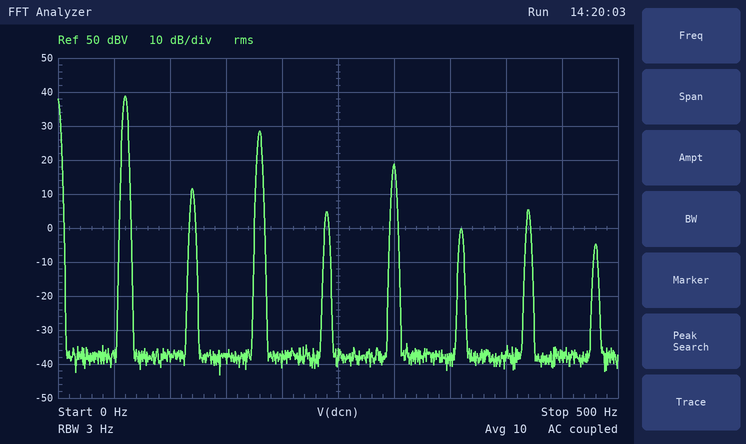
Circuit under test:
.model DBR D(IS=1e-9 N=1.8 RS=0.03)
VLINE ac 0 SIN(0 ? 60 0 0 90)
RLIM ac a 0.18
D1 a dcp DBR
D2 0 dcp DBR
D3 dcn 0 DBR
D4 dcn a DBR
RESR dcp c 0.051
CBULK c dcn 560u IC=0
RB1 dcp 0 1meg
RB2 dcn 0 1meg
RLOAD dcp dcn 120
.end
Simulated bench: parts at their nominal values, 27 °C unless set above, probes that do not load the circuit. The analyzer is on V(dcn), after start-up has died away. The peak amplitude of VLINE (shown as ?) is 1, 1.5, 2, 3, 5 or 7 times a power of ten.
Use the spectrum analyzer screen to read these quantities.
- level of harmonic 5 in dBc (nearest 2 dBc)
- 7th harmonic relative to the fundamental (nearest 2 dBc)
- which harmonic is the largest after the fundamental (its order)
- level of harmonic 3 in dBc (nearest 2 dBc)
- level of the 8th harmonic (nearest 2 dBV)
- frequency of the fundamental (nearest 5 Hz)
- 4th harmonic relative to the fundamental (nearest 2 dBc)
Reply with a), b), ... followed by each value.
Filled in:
a) -20 dBc
b) -34 dBc
c) 3
d) -10 dBc
e) -4 dBV
f) 60 Hz
g) -34 dBc
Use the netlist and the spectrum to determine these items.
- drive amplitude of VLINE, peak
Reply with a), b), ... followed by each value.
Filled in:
a) 300 V
